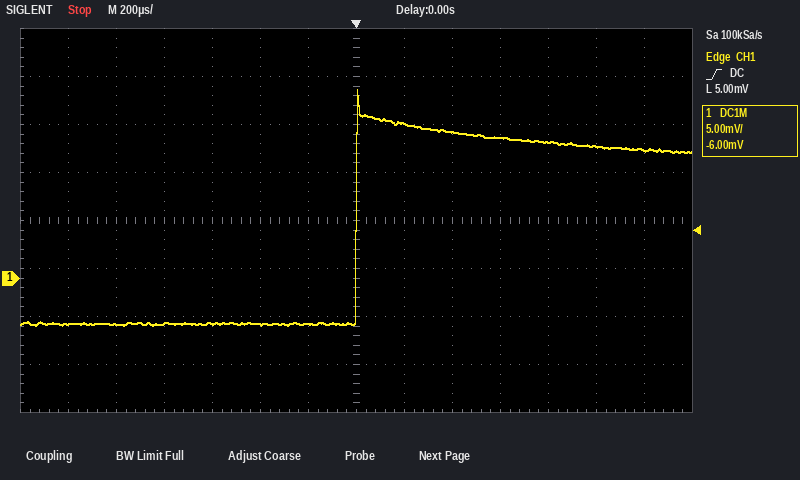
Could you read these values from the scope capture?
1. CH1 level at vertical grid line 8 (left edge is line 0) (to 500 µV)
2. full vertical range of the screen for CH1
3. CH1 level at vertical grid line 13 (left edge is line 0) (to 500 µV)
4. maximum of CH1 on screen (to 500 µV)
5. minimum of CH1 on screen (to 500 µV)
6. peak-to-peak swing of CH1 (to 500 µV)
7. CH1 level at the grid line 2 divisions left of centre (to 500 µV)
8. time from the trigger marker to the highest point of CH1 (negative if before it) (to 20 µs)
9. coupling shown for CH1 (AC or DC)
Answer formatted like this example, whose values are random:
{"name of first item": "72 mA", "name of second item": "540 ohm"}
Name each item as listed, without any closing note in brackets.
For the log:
{"CH1 level at vertical grid line 8 (left edge is line 0)": "16.0 mV", "full vertical range of the screen for CH1": "40 mV", "CH1 level at vertical grid line 13 (left edge is line 0)": "13.5 mV", "maximum of CH1 on screen": "19.5 mV", "minimum of CH1 on screen": "-5.0 mV", "peak-to-peak swing of CH1": "24.5 mV", "CH1 level at the grid line 2 divisions left of centre": "-5.0 mV", "time from the trigger marker to the highest point of CH1 (negative if before it)": "0 µs", "coupling shown for CH1": "DC"}
